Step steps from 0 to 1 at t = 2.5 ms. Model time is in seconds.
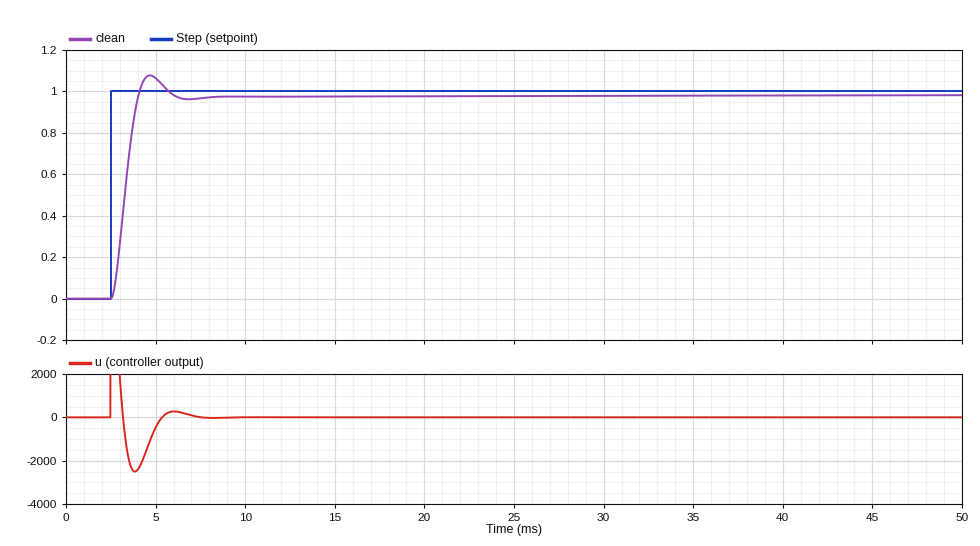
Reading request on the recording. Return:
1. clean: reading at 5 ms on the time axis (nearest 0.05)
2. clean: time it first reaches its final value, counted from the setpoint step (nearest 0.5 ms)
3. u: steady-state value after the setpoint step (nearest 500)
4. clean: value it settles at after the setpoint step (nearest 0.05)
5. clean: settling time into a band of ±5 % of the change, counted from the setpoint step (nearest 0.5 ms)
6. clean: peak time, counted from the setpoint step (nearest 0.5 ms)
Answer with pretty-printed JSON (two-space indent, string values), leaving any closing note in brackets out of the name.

{
  "clean: reading at 5 ms on the time axis": "1.05",
  "clean: time it first reaches its final value, counted from the setpoint step": "1.5 ms",
  "u: steady-state value after the setpoint step": "0",
  "clean: value it settles at after the setpoint step": "1.00",
  "clean: settling time into a band of ±5 % of the change, counted from the setpoint step": "3.0 ms",
  "clean: peak time, counted from the setpoint step": "2.0 ms"
}
